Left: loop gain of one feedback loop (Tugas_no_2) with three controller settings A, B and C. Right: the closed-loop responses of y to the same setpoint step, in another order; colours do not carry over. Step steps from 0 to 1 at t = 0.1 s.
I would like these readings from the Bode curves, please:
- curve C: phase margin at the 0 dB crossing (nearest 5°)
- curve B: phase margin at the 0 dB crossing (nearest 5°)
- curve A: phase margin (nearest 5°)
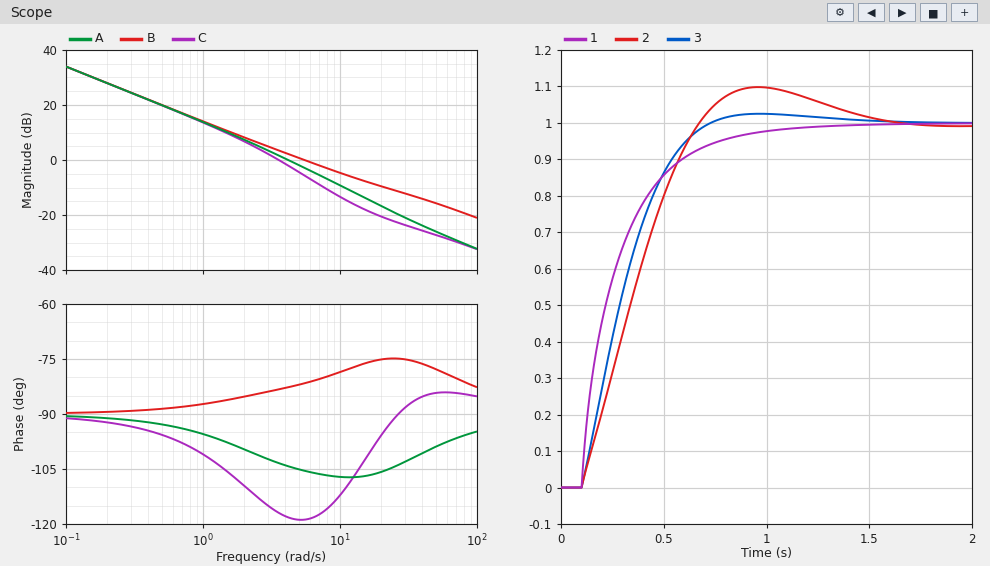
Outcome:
65°
100°
75°
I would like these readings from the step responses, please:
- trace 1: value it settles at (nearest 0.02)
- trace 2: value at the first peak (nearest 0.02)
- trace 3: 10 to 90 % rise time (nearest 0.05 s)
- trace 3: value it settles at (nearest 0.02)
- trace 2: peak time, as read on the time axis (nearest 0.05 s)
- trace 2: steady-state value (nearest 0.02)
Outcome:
1.00
1.10
0.40 s
1.00
0.95 s
1.00
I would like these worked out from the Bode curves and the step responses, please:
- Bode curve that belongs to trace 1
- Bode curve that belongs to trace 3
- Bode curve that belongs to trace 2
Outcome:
B
A
C
